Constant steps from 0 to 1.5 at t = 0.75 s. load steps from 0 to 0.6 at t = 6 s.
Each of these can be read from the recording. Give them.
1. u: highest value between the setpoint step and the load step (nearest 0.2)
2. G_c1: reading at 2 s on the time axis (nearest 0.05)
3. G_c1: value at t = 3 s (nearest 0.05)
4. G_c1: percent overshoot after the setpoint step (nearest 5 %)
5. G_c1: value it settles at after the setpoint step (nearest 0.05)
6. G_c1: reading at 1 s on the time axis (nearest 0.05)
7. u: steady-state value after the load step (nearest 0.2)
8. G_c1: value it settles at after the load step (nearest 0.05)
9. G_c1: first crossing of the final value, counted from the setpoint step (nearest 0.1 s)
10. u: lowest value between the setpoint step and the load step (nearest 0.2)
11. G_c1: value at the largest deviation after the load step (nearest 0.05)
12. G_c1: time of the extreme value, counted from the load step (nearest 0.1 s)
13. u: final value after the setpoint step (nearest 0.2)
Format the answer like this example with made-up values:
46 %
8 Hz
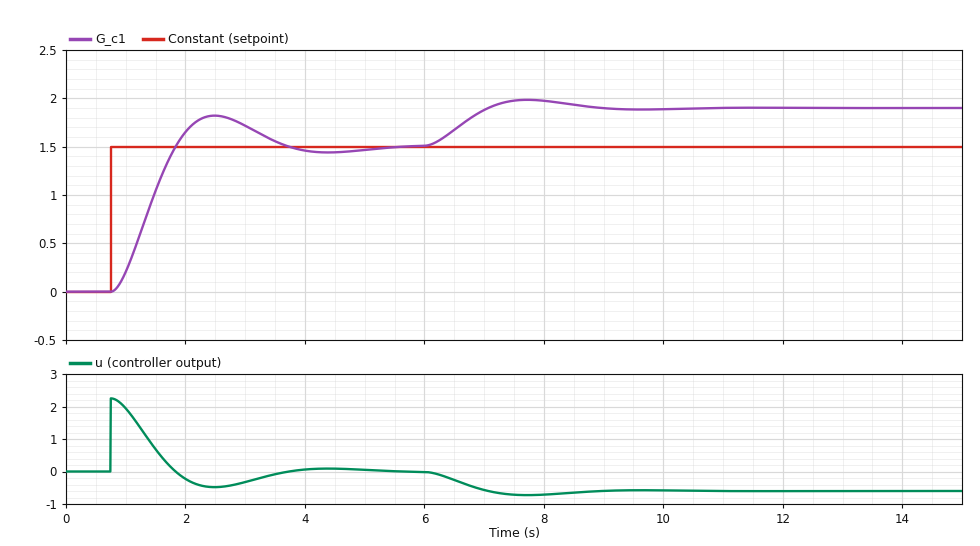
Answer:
2.2
1.65
1.70
20 %
1.50
0.20
-0.6
1.90
1.1 s
-0.4
2.00
1.7 s
0.0
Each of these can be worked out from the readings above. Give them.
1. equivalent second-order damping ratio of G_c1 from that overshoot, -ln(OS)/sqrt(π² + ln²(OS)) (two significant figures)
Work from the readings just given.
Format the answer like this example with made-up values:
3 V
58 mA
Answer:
0.46
